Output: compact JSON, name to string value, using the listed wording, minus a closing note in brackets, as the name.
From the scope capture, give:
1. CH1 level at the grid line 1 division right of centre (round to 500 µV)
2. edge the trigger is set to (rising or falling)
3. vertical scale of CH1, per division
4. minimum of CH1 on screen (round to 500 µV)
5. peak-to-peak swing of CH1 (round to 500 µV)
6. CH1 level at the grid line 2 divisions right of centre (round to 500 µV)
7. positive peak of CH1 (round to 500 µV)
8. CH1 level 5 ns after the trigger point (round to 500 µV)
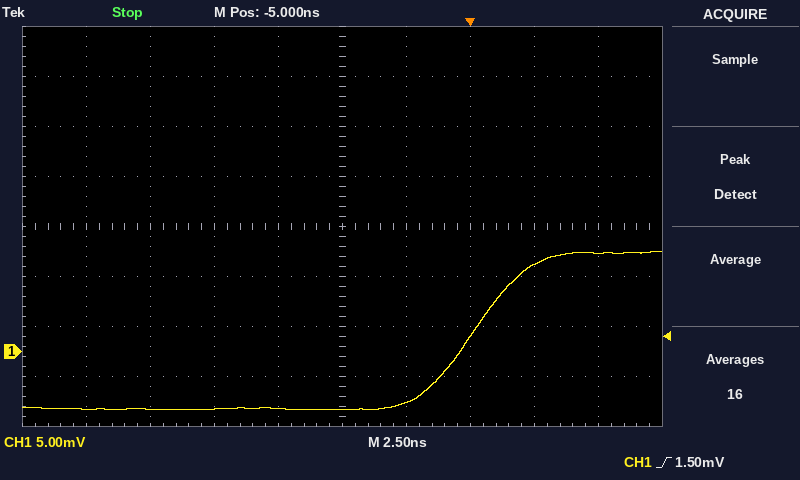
{"CH1 level at the grid line 1 division right of centre": "-5.0 mV", "edge the trigger is set to": "rising", "vertical scale of CH1, per division": "5 mV", "minimum of CH1 on screen": "-6.0 mV", "peak-to-peak swing of CH1": "16.0 mV", "CH1 level at the grid line 2 divisions right of centre": "1.5 mV", "positive peak of CH1": "10.0 mV", "CH1 level 5 ns after the trigger point": "10.0 mV"}
